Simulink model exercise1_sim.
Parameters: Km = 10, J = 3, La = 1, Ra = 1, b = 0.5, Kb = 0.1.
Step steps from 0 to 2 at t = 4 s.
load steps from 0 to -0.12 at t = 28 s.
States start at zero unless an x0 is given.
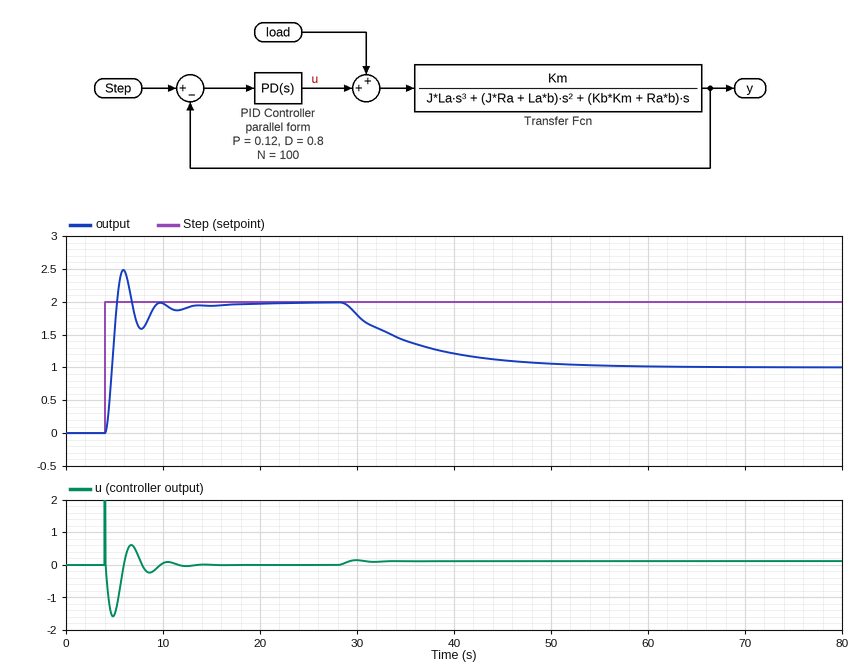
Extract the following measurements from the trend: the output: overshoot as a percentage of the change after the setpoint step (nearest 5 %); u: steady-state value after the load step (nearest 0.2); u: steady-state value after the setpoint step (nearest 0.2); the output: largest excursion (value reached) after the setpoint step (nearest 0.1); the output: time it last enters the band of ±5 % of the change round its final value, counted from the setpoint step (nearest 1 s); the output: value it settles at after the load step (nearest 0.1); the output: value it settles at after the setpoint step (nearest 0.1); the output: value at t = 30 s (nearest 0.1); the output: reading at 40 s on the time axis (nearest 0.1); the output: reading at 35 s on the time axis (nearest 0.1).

25 %
0.2
0.0
2.5
8 s
1.0
2.0
1.8
1.2
1.4
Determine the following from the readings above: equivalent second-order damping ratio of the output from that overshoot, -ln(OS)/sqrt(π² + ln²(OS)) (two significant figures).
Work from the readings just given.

0.40
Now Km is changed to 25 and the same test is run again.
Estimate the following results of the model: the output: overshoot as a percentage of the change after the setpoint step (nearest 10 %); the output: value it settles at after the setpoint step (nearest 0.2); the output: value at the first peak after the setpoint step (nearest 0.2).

40 %
2.0
2.8
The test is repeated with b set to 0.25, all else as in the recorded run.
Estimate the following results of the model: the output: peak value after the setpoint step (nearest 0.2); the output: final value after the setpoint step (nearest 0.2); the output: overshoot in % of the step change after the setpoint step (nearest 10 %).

2.6
2.0
30 %
